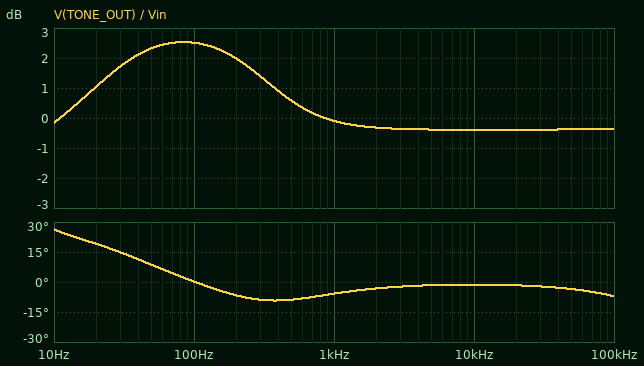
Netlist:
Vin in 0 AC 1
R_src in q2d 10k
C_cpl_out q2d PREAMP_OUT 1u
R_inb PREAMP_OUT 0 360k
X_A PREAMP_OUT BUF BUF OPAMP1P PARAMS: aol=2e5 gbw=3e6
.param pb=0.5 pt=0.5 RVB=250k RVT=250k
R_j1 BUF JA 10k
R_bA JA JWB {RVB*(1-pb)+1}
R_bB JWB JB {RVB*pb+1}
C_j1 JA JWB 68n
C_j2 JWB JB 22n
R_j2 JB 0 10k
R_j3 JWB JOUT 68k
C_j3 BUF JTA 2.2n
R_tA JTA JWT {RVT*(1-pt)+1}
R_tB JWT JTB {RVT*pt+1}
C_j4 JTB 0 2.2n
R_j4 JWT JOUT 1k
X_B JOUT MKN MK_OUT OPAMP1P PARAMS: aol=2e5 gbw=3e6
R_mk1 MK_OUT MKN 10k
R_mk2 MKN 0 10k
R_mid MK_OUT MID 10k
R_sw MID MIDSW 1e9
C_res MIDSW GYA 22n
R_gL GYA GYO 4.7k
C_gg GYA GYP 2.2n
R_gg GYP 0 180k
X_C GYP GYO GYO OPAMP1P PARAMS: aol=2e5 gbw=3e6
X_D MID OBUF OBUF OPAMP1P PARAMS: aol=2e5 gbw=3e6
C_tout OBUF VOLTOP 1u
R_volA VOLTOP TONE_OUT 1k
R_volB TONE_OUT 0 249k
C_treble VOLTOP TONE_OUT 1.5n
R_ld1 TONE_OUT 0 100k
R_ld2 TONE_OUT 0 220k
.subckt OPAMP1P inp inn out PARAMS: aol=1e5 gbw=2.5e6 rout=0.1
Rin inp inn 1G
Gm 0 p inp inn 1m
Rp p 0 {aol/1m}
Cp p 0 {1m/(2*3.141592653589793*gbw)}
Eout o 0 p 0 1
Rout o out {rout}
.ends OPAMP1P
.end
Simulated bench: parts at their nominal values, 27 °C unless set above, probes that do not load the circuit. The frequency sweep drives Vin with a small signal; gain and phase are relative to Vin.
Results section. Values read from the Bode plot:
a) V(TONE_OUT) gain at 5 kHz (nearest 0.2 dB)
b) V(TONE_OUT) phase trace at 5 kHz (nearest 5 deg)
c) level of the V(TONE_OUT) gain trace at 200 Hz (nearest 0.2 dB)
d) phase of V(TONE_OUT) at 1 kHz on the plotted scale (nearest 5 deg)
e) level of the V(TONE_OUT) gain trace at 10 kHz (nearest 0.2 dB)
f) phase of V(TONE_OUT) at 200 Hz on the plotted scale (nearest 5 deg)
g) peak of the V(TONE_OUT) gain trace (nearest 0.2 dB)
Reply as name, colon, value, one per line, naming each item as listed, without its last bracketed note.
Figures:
V(TONE_OUT) gain at 5 kHz: -0.4 dB
V(TONE_OUT) phase trace at 5 kHz: 0 deg
level of the V(TONE_OUT) gain trace at 200 Hz: 2.0 dB
phase of V(TONE_OUT) at 1 kHz on the plotted scale: -5 deg
level of the V(TONE_OUT) gain trace at 10 kHz: -0.4 dB
phase of V(TONE_OUT) at 200 Hz on the plotted scale: -5 deg
peak of the V(TONE_OUT) gain trace: 2.6 dB
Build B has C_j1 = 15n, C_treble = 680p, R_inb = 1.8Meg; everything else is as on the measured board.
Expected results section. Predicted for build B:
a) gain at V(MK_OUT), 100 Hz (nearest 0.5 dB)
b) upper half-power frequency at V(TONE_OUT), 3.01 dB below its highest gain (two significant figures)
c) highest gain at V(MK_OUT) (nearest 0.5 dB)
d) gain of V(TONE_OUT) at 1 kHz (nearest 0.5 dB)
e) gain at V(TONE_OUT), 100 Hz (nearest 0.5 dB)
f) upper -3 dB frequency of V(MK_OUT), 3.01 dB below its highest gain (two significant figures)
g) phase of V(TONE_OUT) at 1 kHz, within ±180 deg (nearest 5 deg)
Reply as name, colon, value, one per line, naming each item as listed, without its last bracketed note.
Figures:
gain at V(MK_OUT), 100 Hz: -1.0 dB
upper half-power frequency at V(TONE_OUT), 3.01 dB below its highest gain: 1.1 MHz
highest gain at V(MK_OUT): 0 dB
gain of V(TONE_OUT) at 1 kHz: -0.5 dB
gain at V(TONE_OUT), 100 Hz: -1.5 dB
upper -3 dB frequency of V(MK_OUT), 3.01 dB below its highest gain: 1.3 MHz
phase of V(TONE_OUT) at 1 kHz, within ±180 deg: 5 deg
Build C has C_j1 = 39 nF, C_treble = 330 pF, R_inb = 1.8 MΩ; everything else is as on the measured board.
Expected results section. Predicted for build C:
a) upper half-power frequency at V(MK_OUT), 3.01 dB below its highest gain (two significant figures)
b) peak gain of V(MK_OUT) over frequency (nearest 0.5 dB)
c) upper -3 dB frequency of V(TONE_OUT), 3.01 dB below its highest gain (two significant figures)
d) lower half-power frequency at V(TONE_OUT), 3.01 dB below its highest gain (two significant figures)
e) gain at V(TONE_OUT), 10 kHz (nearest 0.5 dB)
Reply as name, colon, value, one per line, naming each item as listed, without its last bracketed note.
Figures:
upper half-power frequency at V(MK_OUT), 3.01 dB below its highest gain: 790 kHz
peak gain of V(MK_OUT) over frequency: 1.5 dB
upper -3 dB frequency of V(TONE_OUT), 3.01 dB below its highest gain: 740 kHz
lower half-power frequency at V(TONE_OUT), 3.01 dB below its highest gain: 4.7 Hz
gain at V(TONE_OUT), 10 kHz: 0 dB
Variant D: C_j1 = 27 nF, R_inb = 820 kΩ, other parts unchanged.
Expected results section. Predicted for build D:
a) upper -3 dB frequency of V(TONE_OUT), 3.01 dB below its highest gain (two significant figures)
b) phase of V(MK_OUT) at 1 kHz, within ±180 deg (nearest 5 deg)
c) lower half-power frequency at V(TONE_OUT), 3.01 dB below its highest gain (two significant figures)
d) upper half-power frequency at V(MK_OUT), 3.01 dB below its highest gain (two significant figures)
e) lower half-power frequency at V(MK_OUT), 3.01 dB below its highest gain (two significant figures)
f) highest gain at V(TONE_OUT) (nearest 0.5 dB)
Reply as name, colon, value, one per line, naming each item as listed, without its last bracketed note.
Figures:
upper -3 dB frequency of V(TONE_OUT), 3.01 dB below its highest gain: 1.0 MHz
phase of V(MK_OUT) at 1 kHz, within ±180 deg: 0 deg
lower half-power frequency at V(TONE_OUT), 3.01 dB below its highest gain: 3.4 Hz
upper half-power frequency at V(MK_OUT), 3.01 dB below its highest gain: 1.1 MHz
lower half-power frequency at V(MK_OUT), 3.01 dB below its highest gain: 220 mHz
highest gain at V(TONE_OUT): 0.5 dB
